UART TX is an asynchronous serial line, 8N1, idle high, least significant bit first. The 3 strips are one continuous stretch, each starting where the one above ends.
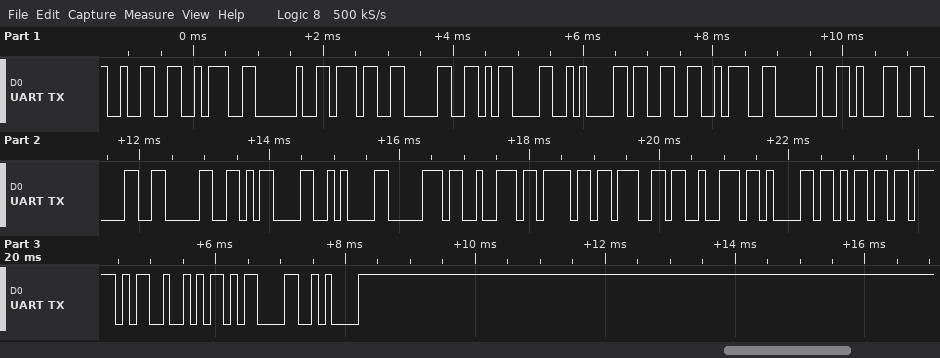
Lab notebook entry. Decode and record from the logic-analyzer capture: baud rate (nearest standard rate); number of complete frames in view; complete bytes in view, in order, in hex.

9600 baud
26
32 3A 20 37 30 0D 0A 33 3A 20 31 30 30 0D 0A 70 72 6F 67 72 61 6D 5F 52 0D 0A
